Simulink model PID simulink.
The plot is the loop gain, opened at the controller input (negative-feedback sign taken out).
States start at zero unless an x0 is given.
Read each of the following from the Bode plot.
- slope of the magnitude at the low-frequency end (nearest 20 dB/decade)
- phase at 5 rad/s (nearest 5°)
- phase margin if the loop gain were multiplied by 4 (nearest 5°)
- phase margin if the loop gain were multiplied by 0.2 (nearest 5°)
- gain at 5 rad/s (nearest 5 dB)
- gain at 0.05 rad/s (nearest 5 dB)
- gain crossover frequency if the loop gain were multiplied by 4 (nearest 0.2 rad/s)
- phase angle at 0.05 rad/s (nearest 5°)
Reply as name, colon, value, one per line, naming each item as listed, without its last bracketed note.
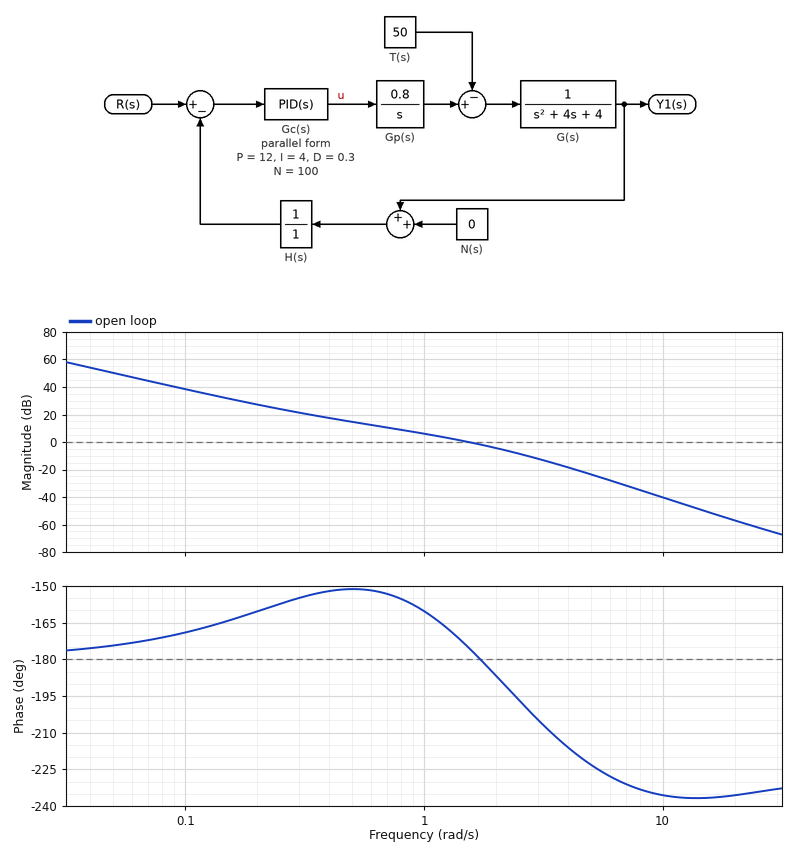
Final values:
slope of the magnitude at the low-frequency end: -40 dB/decade
phase at 5 rad/s: -225°
phase margin if the loop gain were multiplied by 4: -25°
phase margin if the loop gain were multiplied by 0.2: 30°
gain at 5 rad/s: -25 dB
gain at 0.05 rad/s: 50 dB
gain crossover frequency if the loop gain were multiplied by 4: 3.0 rad/s
phase angle at 0.05 rad/s: -175°
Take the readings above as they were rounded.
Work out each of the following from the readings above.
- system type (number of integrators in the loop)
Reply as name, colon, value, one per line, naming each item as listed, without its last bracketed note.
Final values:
system type: 2
